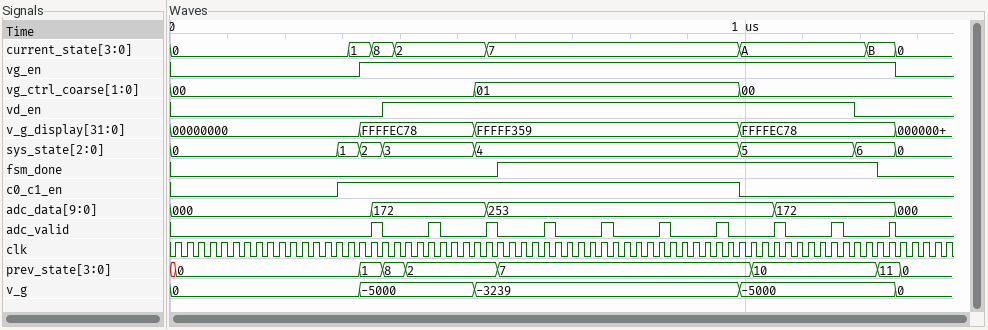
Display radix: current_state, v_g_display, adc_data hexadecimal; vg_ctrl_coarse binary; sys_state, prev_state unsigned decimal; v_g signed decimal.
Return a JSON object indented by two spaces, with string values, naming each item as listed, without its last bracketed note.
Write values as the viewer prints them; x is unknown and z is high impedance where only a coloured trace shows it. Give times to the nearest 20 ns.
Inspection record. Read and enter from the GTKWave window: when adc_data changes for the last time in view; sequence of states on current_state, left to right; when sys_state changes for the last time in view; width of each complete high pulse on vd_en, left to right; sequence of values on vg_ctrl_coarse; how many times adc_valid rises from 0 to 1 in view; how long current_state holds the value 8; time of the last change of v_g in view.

{
  "when adc_data changes for the last time in view": "1260 ns",
  "sequence of states on current_state, left to right": "0, 1, 8, 2, 7, A, B, 0",
  "when sys_state changes for the last time in view": "1260 ns",
  "width of each complete high pulse on vd_en, left to right": "820 ns",
  "sequence of values on vg_ctrl_coarse": "00, 01, 00",
  "how many times adc_valid rises from 0 to 1 in view": "10",
  "how long current_state holds the value 8": "40 ns",
  "time of the last change of v_g in view": "1260 ns"
}
